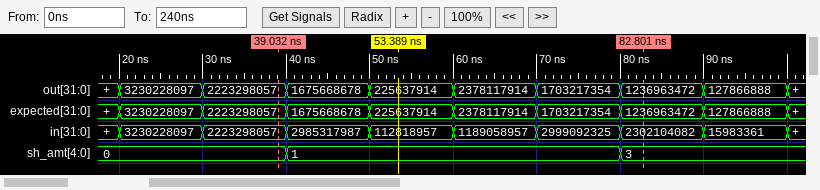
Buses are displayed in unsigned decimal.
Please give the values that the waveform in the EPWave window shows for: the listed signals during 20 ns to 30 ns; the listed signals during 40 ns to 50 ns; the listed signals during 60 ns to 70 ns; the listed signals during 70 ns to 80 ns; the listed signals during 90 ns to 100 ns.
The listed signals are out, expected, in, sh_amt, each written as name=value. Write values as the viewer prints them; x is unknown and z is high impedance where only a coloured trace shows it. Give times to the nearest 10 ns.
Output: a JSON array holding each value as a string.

["out=3230228097, expected=3230228097, in=3230228097, sh_amt=0", "out=1675668678, expected=1675668678, in=2985317987, sh_amt=1", "out=2378117914, expected=2378117914, in=1189058957, sh_amt=1", "out=1703217354, expected=1703217354, in=2999092325, sh_amt=1", "out=127866888, expected=127866888, in=15983361, sh_amt=3"]
